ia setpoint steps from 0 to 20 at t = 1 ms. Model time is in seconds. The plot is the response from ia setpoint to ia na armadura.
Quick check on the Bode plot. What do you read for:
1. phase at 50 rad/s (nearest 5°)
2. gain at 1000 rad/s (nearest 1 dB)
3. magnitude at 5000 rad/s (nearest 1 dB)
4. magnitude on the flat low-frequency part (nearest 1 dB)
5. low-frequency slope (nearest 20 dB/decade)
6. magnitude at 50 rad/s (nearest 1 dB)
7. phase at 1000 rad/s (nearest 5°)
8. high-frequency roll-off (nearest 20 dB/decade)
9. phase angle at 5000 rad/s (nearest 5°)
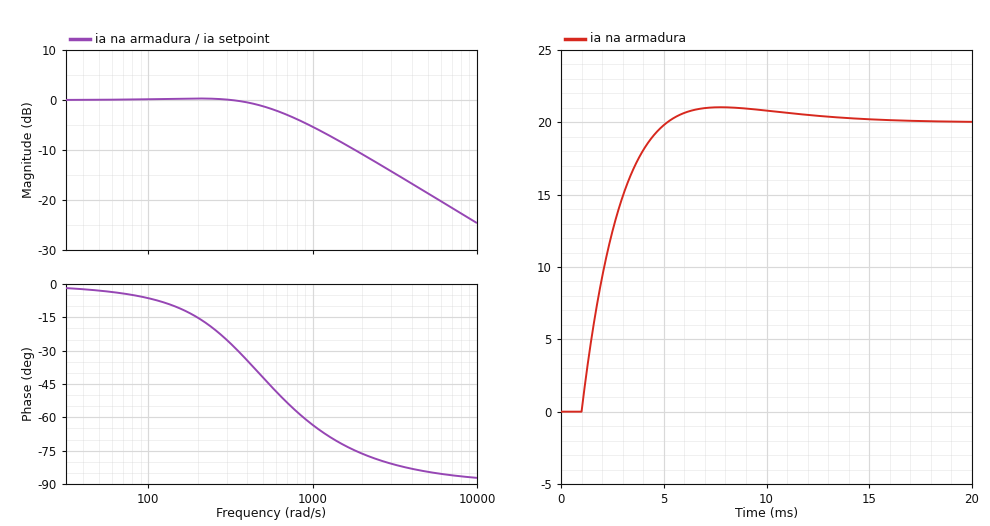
-5°
-5 dB
-19 dB
0 dB
0 dB/decade
0 dB
-65°
-20 dB/decade
-85°
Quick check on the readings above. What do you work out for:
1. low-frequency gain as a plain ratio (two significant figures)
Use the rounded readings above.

1.0
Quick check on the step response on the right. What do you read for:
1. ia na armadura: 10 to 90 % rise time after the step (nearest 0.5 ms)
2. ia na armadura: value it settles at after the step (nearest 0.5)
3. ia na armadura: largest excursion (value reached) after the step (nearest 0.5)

3.0 ms
20.0
21.0
